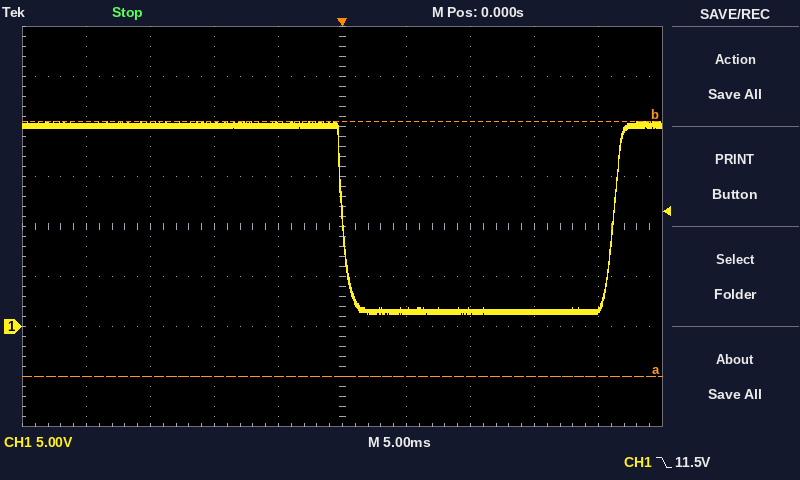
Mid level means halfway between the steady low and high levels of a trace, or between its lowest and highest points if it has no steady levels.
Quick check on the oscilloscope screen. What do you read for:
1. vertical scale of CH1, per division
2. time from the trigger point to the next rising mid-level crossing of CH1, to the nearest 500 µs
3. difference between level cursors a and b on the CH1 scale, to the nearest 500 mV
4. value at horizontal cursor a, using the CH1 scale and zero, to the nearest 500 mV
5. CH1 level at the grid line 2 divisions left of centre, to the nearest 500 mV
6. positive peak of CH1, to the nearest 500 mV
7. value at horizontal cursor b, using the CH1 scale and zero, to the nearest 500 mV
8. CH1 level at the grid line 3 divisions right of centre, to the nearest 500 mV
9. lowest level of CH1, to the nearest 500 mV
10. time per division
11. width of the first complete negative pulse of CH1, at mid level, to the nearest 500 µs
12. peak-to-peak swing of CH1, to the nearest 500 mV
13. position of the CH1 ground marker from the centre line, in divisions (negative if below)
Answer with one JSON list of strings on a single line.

["5 V", "21.0 ms", "25.5 V", "-5.0 V", "20.0 V", "20.5 V", "20.5 V", "1.5 V", "1.5 V", "5 ms", "21.0 ms", "19.0 V", "-2.0 div"]
